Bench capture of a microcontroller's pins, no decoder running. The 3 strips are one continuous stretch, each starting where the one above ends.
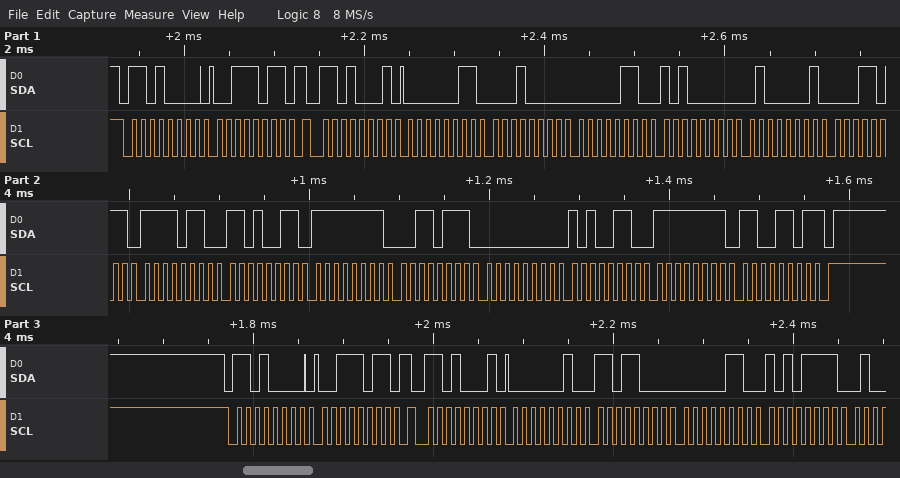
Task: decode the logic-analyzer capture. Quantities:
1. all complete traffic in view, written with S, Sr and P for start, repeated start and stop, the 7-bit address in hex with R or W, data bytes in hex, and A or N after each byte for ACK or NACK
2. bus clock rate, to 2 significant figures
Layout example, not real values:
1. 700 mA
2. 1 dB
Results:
1. S 68W A 3B A Sr 68R A 03 A 10 A 06 A A0 A 41 A 1B A F6 A D3 A FF A 37 A 00 A A6 A FF A CD N P S 68W A 3B A Sr 68R A 02 A D8 A 06 A AF A
2. 100 kHz
